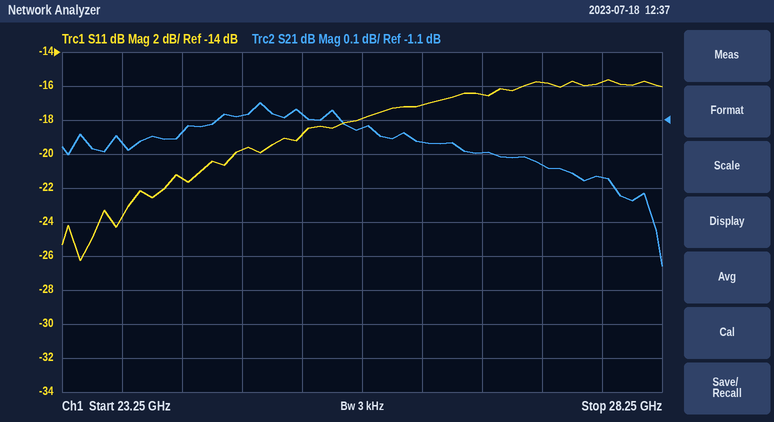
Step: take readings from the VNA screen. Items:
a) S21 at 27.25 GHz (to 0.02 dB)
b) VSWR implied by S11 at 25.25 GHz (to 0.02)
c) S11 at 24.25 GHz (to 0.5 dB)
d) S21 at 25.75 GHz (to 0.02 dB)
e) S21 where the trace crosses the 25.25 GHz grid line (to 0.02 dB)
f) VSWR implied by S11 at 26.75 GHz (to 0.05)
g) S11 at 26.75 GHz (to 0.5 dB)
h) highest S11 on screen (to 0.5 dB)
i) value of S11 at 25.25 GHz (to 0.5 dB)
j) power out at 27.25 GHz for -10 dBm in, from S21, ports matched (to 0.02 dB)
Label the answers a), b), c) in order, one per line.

a) -1.24 dB
b) 1.26
c) -21.5 dB
d) -1.12 dB
e) -1.08 dB
f) 1.35
g) -16.5 dB
h) -15.5 dB
i) -19.0 dB
j) -11.24 dBm
